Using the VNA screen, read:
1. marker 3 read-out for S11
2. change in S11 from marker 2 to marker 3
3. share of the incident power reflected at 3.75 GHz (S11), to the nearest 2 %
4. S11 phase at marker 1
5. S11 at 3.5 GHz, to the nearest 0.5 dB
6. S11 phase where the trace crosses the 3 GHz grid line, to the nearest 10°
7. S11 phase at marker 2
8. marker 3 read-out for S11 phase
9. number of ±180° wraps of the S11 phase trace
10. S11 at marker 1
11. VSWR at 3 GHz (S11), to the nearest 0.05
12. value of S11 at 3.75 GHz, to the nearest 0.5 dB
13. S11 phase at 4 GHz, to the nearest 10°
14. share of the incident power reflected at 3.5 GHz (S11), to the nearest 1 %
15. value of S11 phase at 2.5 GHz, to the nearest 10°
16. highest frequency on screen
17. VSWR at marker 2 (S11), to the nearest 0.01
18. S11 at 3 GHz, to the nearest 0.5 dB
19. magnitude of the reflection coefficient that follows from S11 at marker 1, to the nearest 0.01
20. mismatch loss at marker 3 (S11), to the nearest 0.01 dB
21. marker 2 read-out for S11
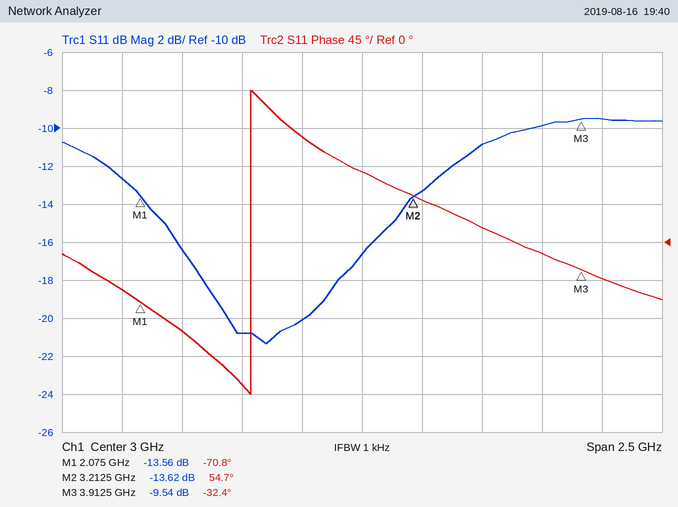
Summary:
-9.54 dB
4.08 dB
10 %
-70.8°
-11.0 dB
80°
54.7°
-32.4°
1
-13.56 dB
1.35
-10.0 dB
-40°
8 %
-170°
4.25 GHz
1.53
-16.5 dB
0.21
0.51 dB
-13.62 dB
